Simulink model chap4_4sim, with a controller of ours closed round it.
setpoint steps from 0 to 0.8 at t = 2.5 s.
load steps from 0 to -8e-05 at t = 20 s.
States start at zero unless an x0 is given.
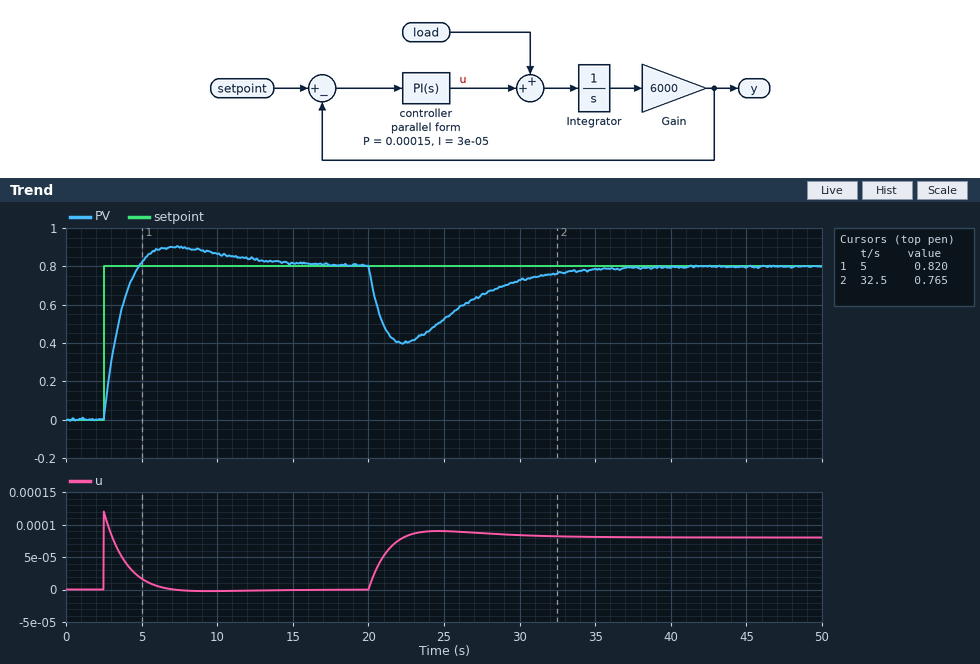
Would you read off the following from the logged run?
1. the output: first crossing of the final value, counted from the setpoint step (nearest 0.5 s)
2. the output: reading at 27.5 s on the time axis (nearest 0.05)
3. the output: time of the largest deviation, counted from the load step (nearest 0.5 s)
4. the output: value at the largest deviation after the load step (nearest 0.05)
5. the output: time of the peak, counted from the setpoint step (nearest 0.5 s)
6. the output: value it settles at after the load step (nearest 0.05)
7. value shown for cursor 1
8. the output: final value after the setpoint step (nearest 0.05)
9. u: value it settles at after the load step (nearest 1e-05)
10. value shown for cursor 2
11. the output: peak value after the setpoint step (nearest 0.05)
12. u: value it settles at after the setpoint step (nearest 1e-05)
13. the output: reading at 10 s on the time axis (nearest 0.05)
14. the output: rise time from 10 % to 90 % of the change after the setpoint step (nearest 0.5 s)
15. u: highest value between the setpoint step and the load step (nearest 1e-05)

2.5 s
0.65
2.5 s
0.40
4.5 s
0.80
0.820
0.80
0.00008
0.765
0.90
0.00000
0.85
1.5 s
0.00012
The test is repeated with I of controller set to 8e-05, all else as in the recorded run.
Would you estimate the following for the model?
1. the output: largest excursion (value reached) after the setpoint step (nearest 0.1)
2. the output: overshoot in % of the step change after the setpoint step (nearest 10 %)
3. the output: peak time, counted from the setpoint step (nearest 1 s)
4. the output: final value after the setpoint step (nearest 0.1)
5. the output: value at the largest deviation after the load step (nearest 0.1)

1.0
20 %
3 s
0.8
0.5
